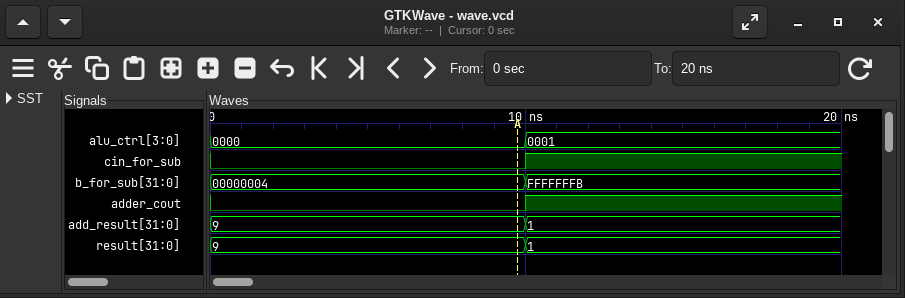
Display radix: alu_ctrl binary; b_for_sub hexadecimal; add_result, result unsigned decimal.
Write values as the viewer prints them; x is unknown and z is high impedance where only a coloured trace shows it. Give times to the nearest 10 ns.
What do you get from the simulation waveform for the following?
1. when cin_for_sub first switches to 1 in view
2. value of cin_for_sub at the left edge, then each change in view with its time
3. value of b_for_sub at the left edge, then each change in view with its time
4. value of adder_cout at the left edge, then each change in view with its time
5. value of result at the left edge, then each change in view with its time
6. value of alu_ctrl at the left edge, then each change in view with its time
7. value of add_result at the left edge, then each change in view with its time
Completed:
10 ns
0, 1 at 10 ns
00000004, FFFFFFFB at 10 ns
0, 1 at 10 ns
9, 1 at 10 ns
0000, 0001 at 10 ns
9, 1 at 10 ns
